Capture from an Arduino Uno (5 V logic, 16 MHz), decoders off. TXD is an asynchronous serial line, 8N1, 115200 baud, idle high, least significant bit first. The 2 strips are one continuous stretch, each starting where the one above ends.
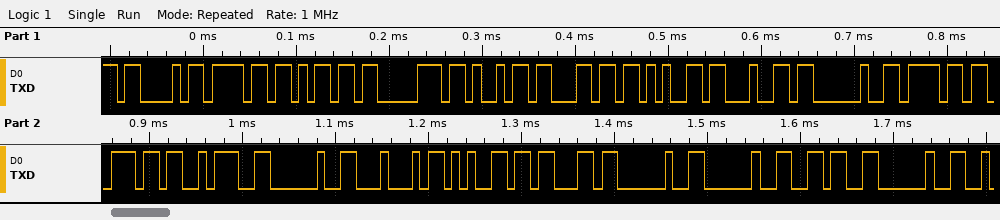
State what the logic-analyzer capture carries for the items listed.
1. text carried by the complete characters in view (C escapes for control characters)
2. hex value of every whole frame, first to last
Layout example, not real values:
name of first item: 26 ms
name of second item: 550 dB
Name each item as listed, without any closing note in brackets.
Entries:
text carried by the complete characters in view: "Compiled on: Dec  6 "
hex value of every whole frame, first to last: 0x43 0x6F 0x6D 0x70 0x69 0x6C 0x65 0x64 0x20 0x6F 0x6E 0x3A 0x20 0x44 0x65 0x63 0x20 0x20 0x36 0x20
